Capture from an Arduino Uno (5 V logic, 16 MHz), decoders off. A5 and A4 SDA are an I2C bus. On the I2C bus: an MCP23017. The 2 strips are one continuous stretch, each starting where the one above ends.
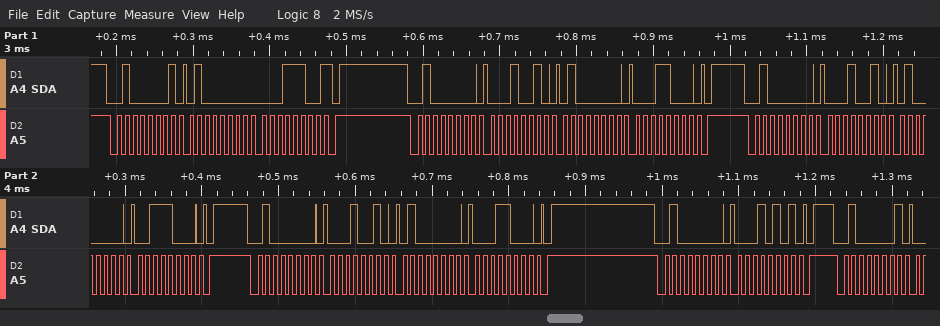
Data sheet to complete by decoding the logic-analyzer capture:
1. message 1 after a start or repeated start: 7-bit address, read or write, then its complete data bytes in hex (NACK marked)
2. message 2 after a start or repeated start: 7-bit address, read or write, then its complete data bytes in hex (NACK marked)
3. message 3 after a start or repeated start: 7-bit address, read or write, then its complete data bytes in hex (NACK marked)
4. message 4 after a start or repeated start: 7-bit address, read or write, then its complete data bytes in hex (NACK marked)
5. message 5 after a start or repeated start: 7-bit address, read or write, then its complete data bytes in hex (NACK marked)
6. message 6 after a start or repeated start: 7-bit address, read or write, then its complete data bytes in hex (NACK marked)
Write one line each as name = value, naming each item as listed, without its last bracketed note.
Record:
message 1 after a start or repeated start: 7-bit address, read or write, then its complete data bytes in hex = 0x20 read: 40 1C NACK
message 2 after a start or repeated start: 7-bit address, read or write, then its complete data bytes in hex = 0x20 write: 12 40 18
message 3 after a start or repeated start: 7-bit address, read or write, then its complete data bytes in hex = 0x20 write: 12 40 38
message 4 after a start or repeated start: 7-bit address, read or write, then its complete data bytes in hex = 0x20 write: 12 40 18
message 5 after a start or repeated start: 7-bit address, read or write, then its complete data bytes in hex = 0x20 write: 15
message 6 after a start or repeated start: 7-bit address, read or write, then its complete data bytes in hex = 0x20 read
